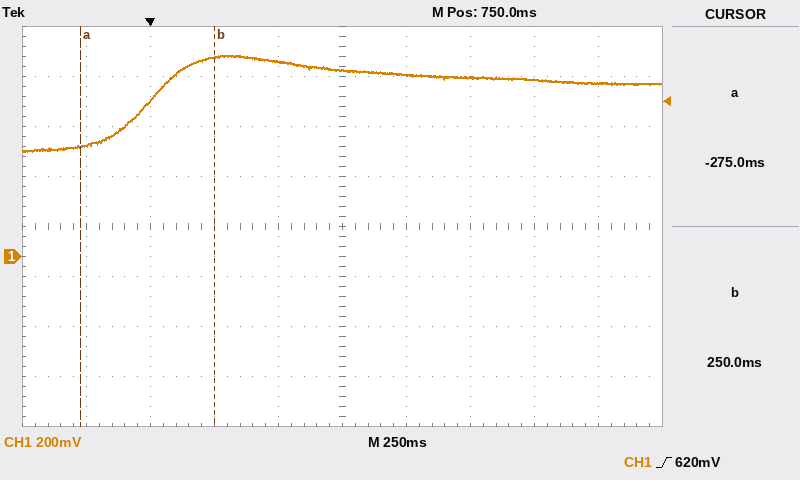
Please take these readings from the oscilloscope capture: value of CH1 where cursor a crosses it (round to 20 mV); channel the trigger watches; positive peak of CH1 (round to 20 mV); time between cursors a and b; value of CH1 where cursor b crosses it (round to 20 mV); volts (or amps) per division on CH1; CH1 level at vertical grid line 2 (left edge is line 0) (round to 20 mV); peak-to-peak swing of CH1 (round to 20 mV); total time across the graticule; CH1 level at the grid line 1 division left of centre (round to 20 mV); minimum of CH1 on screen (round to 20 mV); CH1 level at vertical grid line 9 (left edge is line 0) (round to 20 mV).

440 mV
CH1
800 mV
525 ms
800 mV
200 mV
620 mV
380 mV
2.5 s
780 mV
420 mV
700 mV
